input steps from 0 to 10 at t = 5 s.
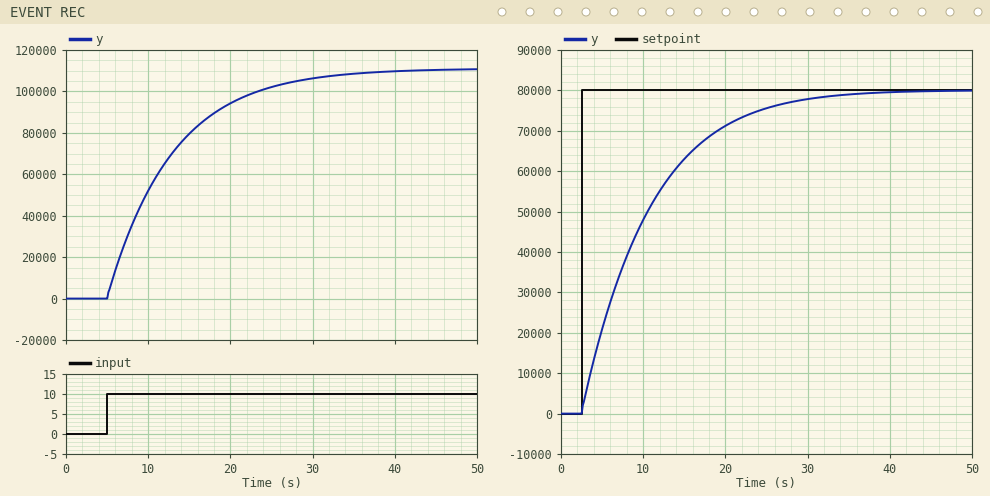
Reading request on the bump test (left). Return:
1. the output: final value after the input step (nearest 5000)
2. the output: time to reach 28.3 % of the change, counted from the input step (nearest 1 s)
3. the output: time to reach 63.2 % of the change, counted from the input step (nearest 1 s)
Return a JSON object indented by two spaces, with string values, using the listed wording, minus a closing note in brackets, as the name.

{
  "the output: final value after the input step": "110000",
  "the output: time to reach 28.3 % of the change, counted from the input step": "3 s",
  "the output: time to reach 63.2 % of the change, counted from the input step": "8 s"
}
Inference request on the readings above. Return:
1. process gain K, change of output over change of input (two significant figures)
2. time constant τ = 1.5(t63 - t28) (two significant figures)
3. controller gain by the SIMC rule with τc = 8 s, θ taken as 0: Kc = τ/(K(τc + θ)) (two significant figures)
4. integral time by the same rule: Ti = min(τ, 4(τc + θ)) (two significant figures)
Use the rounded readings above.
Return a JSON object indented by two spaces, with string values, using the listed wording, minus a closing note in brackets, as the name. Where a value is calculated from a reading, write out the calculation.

{
  "process gain K, change of output over change of input": "(110000 - 0) / 10 = 11000",
  "time constant τ = 1.5(t63 - t28)": "1.5 × (8 - 3) = 7.5 s",
  "controller gain by the SIMC rule with τc = 8 s, θ taken as 0: Kc = τ/(K(τc + θ))": "7.5 / (11000 × (8 + 0)) = 0.000085",
  "integral time by the same rule: Ti = min(τ, 4(τc + θ))": "min(7.5, 4 × (8 + 0)) = 7.5 s"
}
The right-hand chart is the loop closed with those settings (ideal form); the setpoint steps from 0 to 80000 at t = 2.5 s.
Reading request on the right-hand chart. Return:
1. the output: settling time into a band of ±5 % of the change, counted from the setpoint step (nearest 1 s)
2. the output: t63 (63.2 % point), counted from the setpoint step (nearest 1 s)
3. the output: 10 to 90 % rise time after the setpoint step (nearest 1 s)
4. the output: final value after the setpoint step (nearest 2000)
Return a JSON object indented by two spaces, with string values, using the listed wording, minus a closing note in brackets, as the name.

{
  "the output: settling time into a band of ±5 % of the change, counted from the setpoint step": "23 s",
  "the output: t63 (63.2 % point), counted from the setpoint step": "8 s",
  "the output: 10 to 90 % rise time after the setpoint step": "17 s",
  "the output: final value after the setpoint step": "80000"
}
